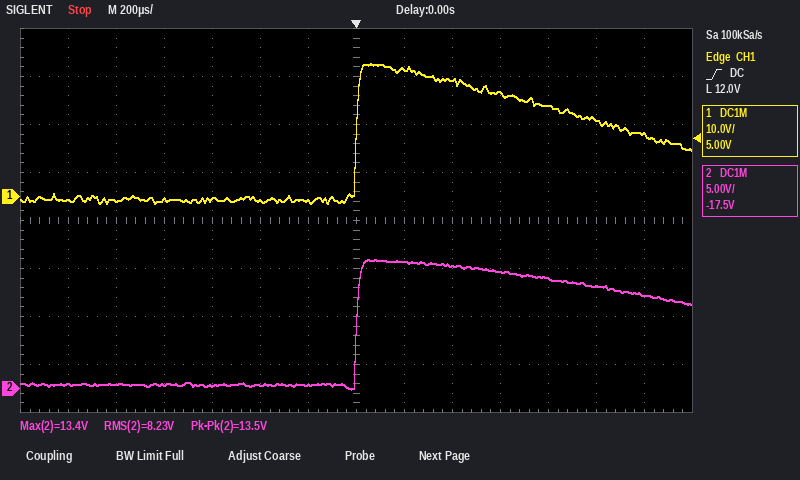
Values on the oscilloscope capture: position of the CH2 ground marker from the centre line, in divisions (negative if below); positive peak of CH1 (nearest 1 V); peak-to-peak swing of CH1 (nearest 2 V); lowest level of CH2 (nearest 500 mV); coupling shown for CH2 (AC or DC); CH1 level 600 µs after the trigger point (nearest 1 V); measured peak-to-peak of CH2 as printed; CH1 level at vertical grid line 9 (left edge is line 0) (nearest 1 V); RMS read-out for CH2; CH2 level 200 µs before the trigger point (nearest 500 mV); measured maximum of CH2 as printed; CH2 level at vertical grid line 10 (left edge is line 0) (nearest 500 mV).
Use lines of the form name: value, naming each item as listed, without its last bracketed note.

position of the CH2 ground marker from the centre line, in divisions: -3.5 div
positive peak of CH1: 28 V
peak-to-peak swing of CH1: 30 V
lowest level of CH2: 0.0 V
coupling shown for CH2: DC
CH1 level 600 µs after the trigger point: 22 V
measured peak-to-peak of CH2 as printed: 13.5 V
CH1 level at vertical grid line 9 (left edge is line 0): 24 V
RMS read-out for CH2: 8.23 V
CH2 level 200 µs before the trigger point: 500 mV
measured maximum of CH2 as printed: 13.4 V
CH2 level at vertical grid line 10 (left edge is line 0): 12.0 V
